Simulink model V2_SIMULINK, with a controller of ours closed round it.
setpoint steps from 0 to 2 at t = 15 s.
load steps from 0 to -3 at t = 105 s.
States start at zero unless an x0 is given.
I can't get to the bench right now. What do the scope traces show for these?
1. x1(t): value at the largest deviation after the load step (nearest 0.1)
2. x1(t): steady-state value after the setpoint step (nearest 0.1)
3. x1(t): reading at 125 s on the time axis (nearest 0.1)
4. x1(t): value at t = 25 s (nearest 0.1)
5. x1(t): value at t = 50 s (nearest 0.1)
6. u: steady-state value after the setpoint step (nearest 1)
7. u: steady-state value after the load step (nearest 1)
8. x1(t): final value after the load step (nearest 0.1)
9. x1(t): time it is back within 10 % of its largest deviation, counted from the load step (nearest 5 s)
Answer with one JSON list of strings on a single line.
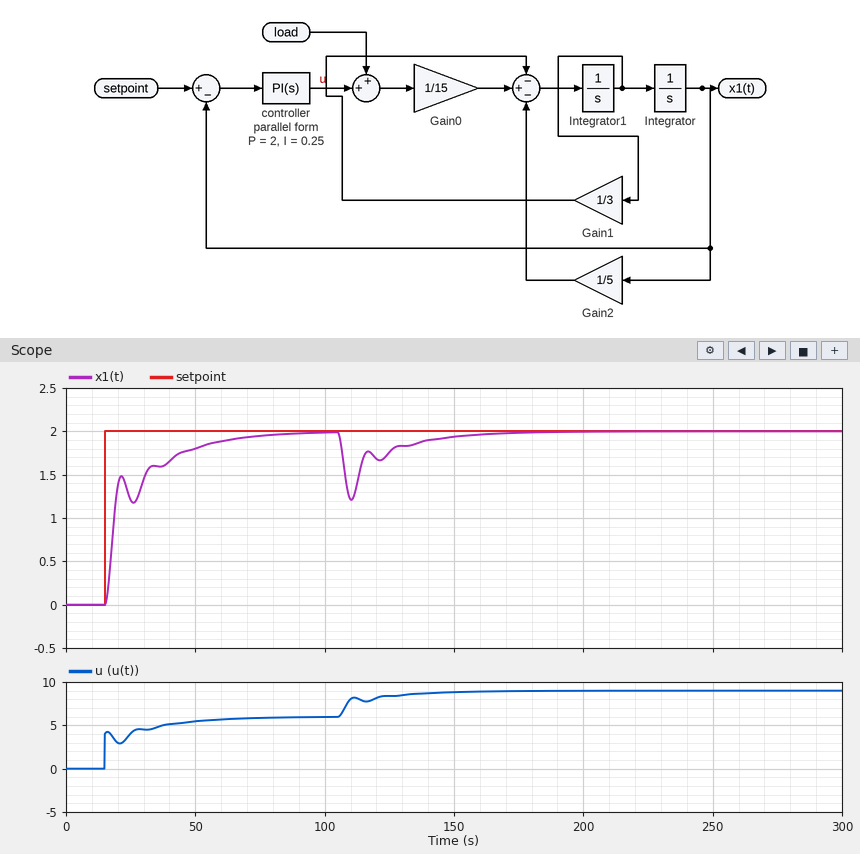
["1.2", "2.0", "1.8", "1.2", "1.8", "6", "9", "2.0", "40 s"]
